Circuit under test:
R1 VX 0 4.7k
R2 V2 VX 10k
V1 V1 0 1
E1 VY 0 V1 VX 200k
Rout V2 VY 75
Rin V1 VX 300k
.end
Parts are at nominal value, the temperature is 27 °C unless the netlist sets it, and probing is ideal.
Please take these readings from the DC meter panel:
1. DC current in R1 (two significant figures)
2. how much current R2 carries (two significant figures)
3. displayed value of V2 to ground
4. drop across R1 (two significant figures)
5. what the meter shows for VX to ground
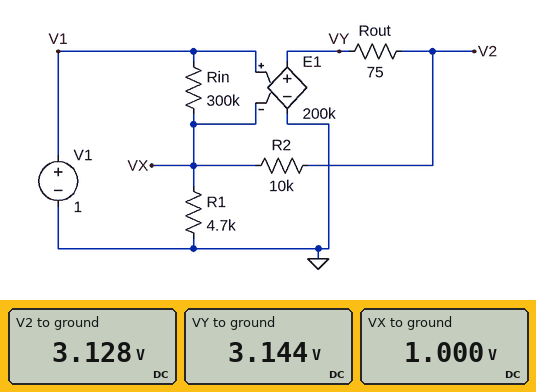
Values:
210 µA
210 µA
3.128 V
1.0 V
1.000 V
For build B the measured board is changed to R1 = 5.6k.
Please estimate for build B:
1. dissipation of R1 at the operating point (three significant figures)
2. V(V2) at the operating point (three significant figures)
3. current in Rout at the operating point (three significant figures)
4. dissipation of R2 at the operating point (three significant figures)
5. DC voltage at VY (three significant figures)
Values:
179 µW
2.79 V
179 µA
319 µW
2.80 V
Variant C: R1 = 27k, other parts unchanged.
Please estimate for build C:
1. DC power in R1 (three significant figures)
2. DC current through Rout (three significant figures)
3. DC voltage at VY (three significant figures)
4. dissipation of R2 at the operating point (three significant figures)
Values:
37.0 µW
37.0 µA
1.37 V
13.7 µW
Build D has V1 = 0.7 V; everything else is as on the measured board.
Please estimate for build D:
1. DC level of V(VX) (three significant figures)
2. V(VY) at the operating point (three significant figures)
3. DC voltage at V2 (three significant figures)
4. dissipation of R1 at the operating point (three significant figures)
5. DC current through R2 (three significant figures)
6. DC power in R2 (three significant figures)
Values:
700 mV
2.20 V
2.19 V
104 µW
149 µA
222 µW
